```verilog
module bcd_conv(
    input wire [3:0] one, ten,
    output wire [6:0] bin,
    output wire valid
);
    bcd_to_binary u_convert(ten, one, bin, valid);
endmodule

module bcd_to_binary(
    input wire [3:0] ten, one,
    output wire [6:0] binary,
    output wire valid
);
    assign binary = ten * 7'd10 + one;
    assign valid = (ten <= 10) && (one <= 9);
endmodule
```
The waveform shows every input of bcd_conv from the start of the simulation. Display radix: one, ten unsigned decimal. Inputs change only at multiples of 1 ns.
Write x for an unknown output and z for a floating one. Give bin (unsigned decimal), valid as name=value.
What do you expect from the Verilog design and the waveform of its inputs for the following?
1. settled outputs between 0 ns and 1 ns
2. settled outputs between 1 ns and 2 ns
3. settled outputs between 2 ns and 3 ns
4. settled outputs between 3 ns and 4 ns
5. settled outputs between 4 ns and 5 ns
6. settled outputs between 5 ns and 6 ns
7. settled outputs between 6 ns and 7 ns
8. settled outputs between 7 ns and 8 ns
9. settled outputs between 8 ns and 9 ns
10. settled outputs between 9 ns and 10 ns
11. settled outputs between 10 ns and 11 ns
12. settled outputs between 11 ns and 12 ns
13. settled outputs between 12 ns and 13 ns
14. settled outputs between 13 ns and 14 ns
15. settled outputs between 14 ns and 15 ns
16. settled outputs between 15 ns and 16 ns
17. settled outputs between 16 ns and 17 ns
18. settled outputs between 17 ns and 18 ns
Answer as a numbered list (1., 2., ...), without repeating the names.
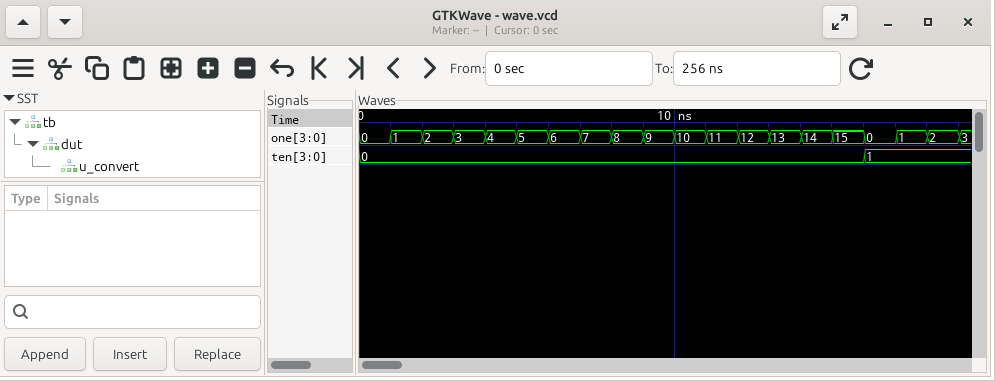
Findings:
1. bin=0, valid=1
2. bin=1, valid=1
3. bin=2, valid=1
4. bin=3, valid=1
5. bin=4, valid=1
6. bin=5, valid=1
7. bin=6, valid=1
8. bin=7, valid=1
9. bin=8, valid=1
10. bin=9, valid=1
11. bin=10, valid=0
12. bin=11, valid=0
13. bin=12, valid=0
14. bin=13, valid=0
15. bin=14, valid=0
16. bin=15, valid=0
17. bin=10, valid=1
18. bin=11, valid=1
